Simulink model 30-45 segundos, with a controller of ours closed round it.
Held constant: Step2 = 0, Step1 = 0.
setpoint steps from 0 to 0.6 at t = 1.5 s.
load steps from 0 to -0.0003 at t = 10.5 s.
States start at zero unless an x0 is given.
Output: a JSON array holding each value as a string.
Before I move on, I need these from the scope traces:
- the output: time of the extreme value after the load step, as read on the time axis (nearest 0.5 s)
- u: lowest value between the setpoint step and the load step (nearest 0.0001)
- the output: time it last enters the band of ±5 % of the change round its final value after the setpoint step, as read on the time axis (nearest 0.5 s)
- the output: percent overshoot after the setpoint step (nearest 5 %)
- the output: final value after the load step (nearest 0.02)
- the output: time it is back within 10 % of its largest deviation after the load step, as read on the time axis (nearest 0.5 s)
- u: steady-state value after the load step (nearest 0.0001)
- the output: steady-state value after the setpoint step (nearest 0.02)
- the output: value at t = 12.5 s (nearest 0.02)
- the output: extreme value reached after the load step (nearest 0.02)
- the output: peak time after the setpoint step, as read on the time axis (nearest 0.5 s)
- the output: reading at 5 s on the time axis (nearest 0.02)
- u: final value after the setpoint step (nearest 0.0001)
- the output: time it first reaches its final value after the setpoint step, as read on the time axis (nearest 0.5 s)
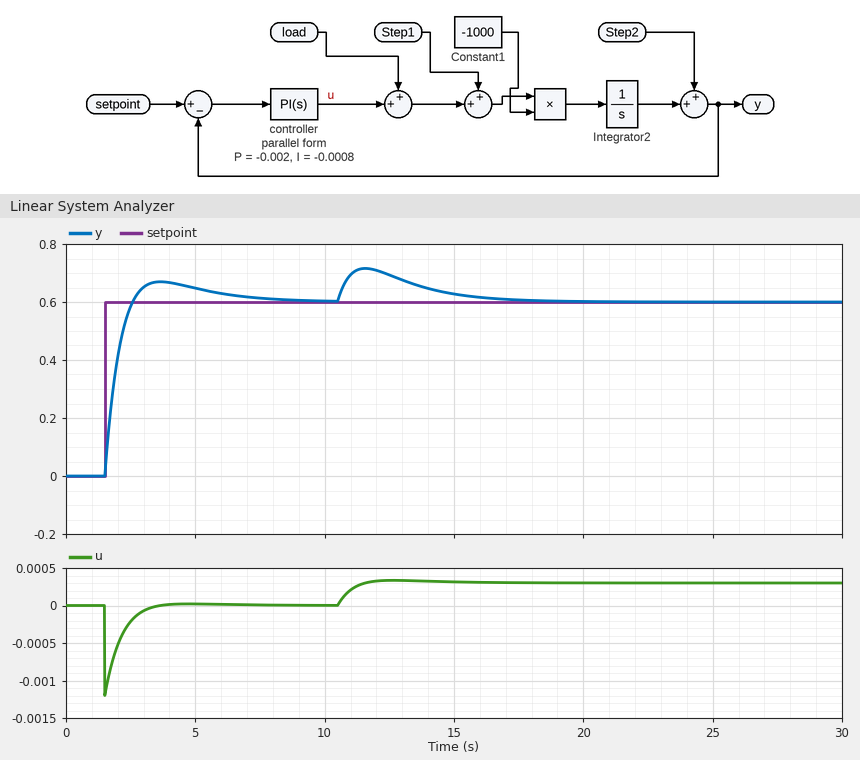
["11.5 s", "-0.0012", "6.0 s", "10 %", "0.60", "16.5 s", "0.0003", "0.60", "0.70", "0.72", "3.5 s", "0.64", "0.0000", "2.5 s"]
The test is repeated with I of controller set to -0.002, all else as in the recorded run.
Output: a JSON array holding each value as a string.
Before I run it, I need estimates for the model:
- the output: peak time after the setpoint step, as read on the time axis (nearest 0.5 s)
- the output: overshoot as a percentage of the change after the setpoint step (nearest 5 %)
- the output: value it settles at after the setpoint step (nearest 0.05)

["3.0 s", "20 %", "0.60"]
